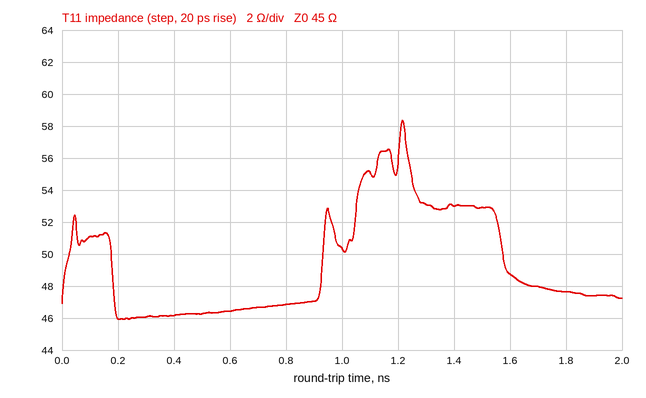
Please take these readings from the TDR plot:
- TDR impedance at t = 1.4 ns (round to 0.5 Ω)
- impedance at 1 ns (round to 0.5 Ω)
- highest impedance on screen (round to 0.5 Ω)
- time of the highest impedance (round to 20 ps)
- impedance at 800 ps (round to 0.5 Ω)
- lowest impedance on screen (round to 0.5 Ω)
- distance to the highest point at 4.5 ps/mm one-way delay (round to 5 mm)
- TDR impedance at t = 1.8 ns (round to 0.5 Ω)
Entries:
53.0 Ω
50.5 Ω
58.5 Ω
1.22 ns
47.0 Ω
46.0 Ω
135 mm
47.5 Ω
